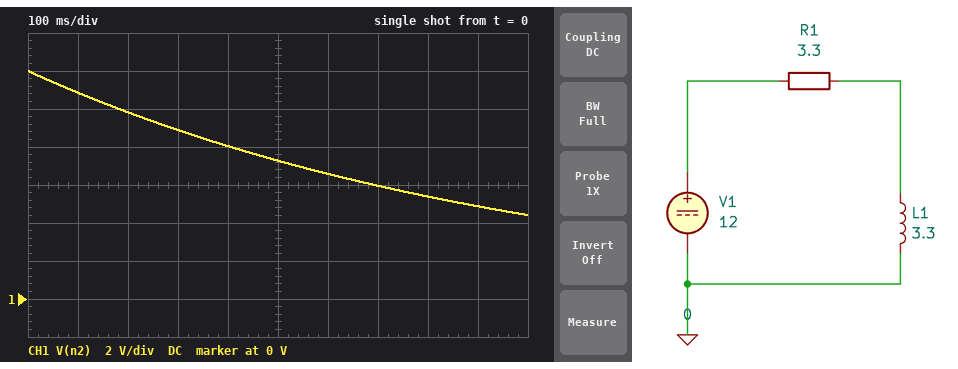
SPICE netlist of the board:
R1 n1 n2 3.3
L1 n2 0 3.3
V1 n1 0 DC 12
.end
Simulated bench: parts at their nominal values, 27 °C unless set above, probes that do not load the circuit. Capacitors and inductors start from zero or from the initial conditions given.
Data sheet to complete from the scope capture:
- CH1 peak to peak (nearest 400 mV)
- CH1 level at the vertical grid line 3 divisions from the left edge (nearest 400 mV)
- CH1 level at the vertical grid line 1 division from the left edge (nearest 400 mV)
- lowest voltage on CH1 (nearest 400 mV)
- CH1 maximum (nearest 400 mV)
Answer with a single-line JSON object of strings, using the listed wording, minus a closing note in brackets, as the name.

{"CH1 peak to peak": "7.6 V", "CH1 level at the vertical grid line 3 divisions from the left edge": "8.8 V", "CH1 level at the vertical grid line 1 division from the left edge": "10.8 V", "lowest voltage on CH1": "4.4 V", "CH1 maximum": "12.0 V"}
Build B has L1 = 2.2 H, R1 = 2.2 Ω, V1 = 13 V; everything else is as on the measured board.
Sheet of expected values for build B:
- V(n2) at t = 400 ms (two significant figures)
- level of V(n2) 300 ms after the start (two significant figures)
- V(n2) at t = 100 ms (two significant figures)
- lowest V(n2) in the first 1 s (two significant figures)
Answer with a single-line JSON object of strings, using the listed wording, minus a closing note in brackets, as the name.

{"V(n2) at t = 400 ms": "8.7 V", "level of V(n2) 300 ms after the start": "9.6 V", "V(n2) at t = 100 ms": "12 V", "lowest V(n2) in the first 1 s": "4.8 V"}
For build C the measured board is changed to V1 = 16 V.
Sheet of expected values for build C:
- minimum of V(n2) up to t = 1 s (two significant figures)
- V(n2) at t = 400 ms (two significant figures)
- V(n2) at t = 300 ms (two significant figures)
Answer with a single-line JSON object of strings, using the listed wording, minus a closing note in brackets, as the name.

{"minimum of V(n2) up to t = 1 s": "5.9 V", "V(n2) at t = 400 ms": "11 V", "V(n2) at t = 300 ms": "12 V"}
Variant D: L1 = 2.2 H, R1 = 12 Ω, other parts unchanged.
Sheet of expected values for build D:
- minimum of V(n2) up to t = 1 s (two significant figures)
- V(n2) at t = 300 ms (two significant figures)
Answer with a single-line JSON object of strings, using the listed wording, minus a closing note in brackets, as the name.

{"minimum of V(n2) up to t = 1 s": "51 mV", "V(n2) at t = 300 ms": "2.3 V"}
